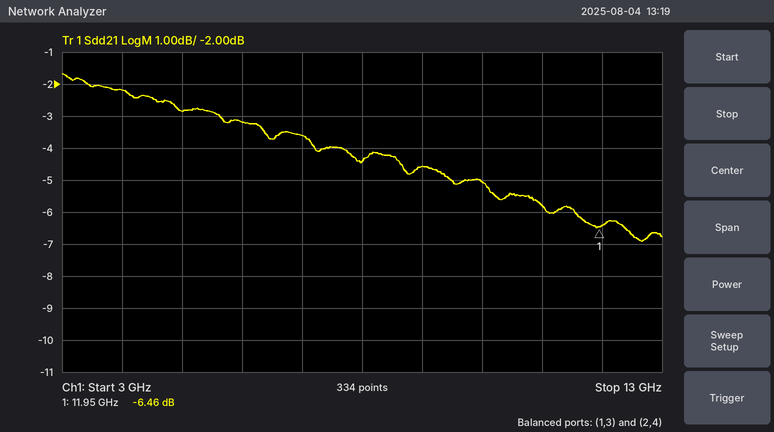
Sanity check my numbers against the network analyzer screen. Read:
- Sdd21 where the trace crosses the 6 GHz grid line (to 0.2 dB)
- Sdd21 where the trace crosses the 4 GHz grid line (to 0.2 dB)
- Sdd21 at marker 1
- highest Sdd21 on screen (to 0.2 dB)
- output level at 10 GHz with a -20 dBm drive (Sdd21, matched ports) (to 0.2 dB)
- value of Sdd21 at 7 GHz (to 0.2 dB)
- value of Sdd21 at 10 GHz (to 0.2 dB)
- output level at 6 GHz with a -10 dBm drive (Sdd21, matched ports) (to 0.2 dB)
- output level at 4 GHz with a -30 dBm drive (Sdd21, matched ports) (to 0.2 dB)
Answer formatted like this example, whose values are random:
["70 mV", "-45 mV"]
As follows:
["-3.2 dB", "-2.2 dB", "-6.46 dB", "-1.6 dB", "-25.0 dBm", "-3.6 dB", "-5.0 dB", "-13.2 dBm", "-32.2 dBm"]
